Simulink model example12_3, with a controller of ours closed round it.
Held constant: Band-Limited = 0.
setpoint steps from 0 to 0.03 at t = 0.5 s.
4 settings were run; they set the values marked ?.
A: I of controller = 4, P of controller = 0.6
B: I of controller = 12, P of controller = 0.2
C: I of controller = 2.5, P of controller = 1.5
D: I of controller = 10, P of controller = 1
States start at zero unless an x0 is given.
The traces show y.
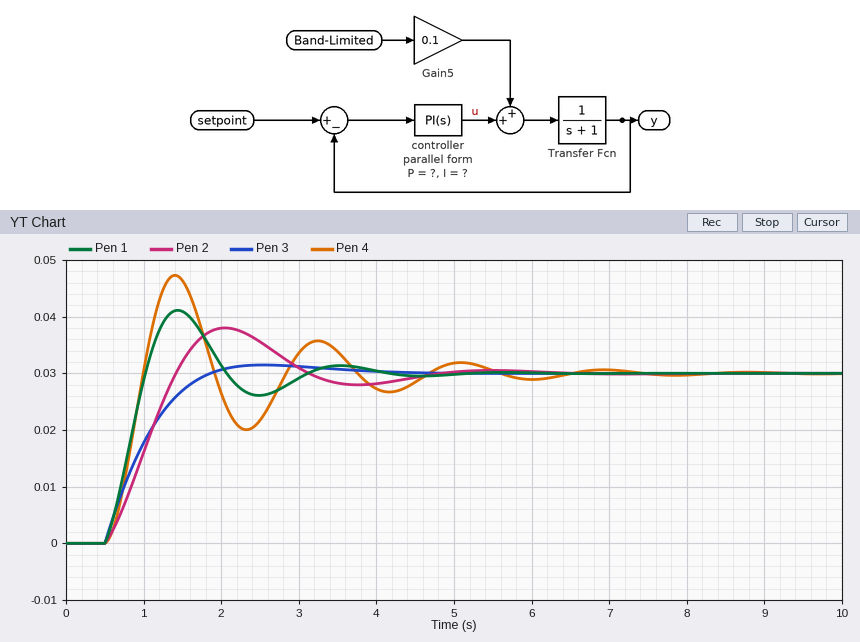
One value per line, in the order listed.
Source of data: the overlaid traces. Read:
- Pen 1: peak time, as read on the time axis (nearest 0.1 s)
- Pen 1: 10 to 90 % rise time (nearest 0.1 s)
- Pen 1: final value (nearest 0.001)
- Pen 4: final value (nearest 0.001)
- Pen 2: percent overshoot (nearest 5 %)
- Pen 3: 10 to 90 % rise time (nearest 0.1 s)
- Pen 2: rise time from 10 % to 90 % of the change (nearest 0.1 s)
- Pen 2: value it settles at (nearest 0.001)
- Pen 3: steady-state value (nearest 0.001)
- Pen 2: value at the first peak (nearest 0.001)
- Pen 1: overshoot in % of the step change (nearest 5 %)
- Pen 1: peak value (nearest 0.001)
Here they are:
1.4 s
0.4 s
0.030
0.030
25 %
0.9 s
0.7 s
0.030
0.030
0.038
35 %
0.041
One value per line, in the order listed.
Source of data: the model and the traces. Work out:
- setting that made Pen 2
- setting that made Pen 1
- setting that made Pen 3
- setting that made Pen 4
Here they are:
A
D
C
B
